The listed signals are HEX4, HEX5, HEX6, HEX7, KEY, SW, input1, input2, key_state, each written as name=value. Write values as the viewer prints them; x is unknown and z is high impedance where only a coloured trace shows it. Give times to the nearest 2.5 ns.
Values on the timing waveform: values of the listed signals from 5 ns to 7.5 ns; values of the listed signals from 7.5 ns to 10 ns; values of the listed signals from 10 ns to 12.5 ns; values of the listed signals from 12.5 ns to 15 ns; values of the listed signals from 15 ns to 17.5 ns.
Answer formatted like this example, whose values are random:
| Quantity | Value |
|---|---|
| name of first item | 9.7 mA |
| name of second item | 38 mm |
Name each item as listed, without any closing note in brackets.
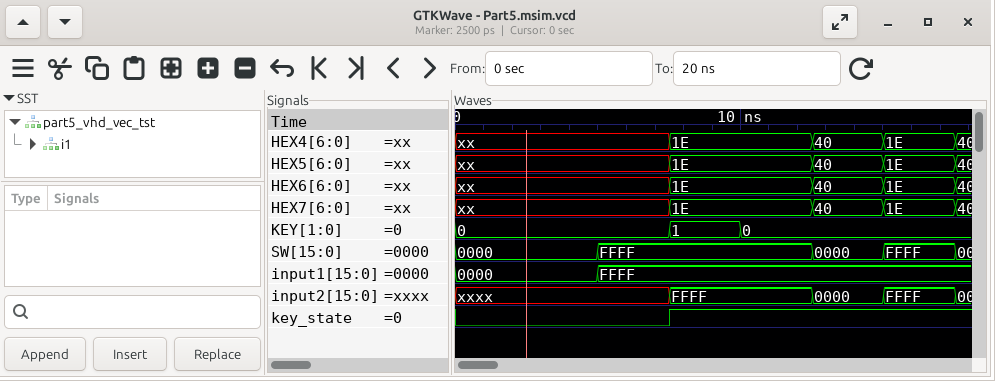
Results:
| Quantity | Value |
|---|---|
| values of the listed signals from 5 ns to 7.5 ns | HEX4=xx, HEX5=xx, HEX6=xx, HEX7=xx, KEY=0, SW=FFFF, input1=FFFF, input2=xxxx, key_state=0 |
| values of the listed signals from 7.5 ns to 10 ns | HEX4=1E, HEX5=1E, HEX6=1E, HEX7=1E, KEY=1, SW=FFFF, input1=FFFF, input2=FFFF, key_state=1 |
| values of the listed signals from 10 ns to 12.5 ns | HEX4=1E, HEX5=1E, HEX6=1E, HEX7=1E, KEY=0, SW=FFFF, input1=FFFF, input2=FFFF, key_state=1 |
| values of the listed signals from 12.5 ns to 15 ns | HEX4=40, HEX5=40, HEX6=40, HEX7=40, KEY=0, SW=0000, input1=FFFF, input2=0000, key_state=1 |
| values of the listed signals from 15 ns to 17.5 ns | HEX4=1E, HEX5=1E, HEX6=1E, HEX7=1E, KEY=0, SW=FFFF, input1=FFFF, input2=FFFF, key_state=1 |
